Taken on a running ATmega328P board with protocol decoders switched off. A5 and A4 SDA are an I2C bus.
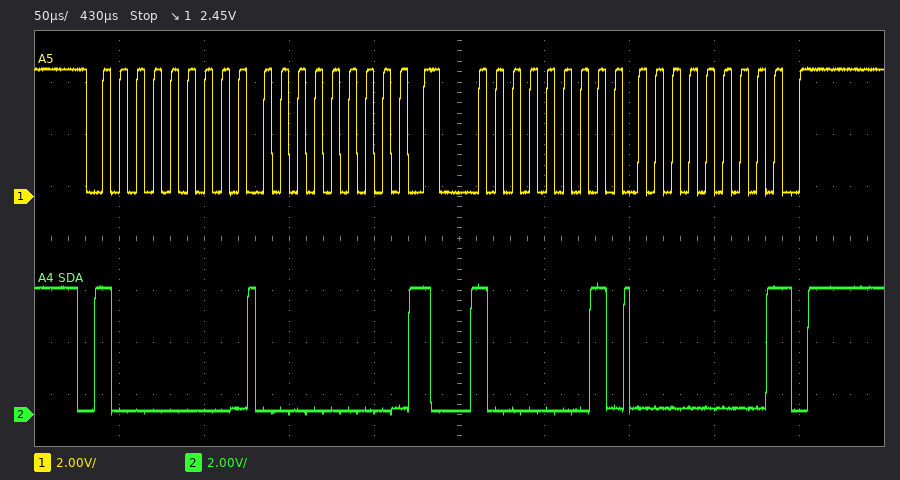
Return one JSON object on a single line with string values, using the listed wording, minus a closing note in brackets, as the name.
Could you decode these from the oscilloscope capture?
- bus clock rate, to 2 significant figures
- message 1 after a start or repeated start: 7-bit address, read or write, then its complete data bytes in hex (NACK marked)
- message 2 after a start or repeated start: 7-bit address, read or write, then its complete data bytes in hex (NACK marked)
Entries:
{"bus clock rate, to 2 significant figures": "100 kHz", "message 1 after a start or repeated start: 7-bit address, read or write, then its complete data bytes in hex": "0x40 write: 00", "message 2 after a start or repeated start: 7-bit address, read or write, then its complete data bytes in hex": "0x40 read: 00 NACK"}
